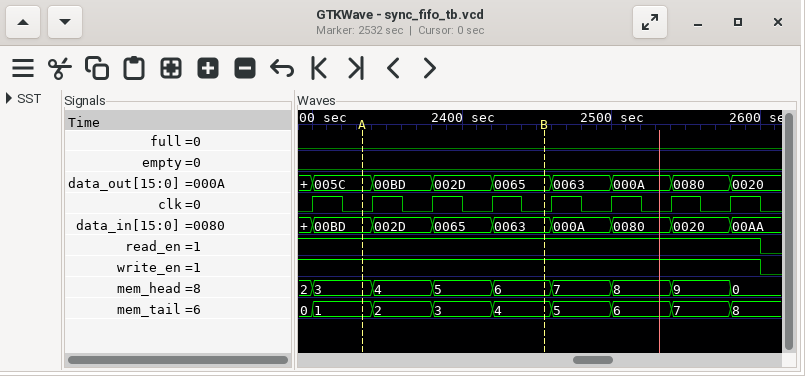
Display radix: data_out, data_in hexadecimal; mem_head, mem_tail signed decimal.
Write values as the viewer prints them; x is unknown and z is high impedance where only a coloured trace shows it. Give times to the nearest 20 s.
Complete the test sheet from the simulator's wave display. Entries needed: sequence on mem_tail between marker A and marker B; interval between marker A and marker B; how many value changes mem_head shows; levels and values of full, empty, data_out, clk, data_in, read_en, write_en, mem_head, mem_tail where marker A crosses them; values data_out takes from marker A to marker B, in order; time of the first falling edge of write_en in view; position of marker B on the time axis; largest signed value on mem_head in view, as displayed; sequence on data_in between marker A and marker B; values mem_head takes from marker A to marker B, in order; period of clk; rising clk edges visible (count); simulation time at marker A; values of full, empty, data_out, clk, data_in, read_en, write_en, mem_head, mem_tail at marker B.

1, 2, 3, 4
120 s
8
full=0, empty=0, data_out=005C, clk=0, data_in=00BD, read_en=1, write_en=1, mem_head=3, mem_tail=1
005C, 00BD, 002D, 0065
2600 s
2460 s
9
00BD, 002D, 0065, 0063
3, 4, 5, 6
40 s
8
2340 s
full=0, empty=0, data_out=0065, clk=0, data_in=0063, read_en=1, write_en=1, mem_head=6, mem_tail=4
